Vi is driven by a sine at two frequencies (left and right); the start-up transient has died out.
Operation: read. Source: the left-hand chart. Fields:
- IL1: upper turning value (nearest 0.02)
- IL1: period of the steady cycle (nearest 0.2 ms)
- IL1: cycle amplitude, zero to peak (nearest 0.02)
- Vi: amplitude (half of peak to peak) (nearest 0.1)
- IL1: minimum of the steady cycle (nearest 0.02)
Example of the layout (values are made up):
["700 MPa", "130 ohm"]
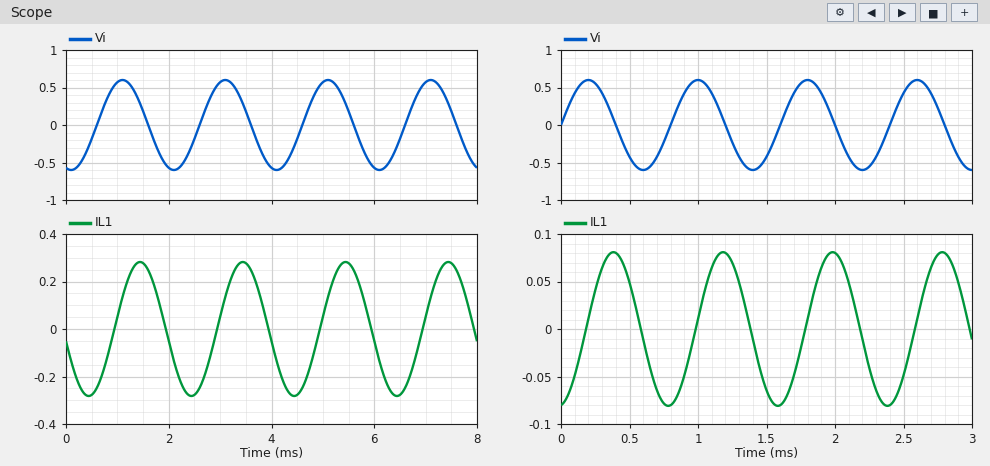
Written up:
["0.28", "2.0 ms", "0.28", "0.6", "-0.28"]
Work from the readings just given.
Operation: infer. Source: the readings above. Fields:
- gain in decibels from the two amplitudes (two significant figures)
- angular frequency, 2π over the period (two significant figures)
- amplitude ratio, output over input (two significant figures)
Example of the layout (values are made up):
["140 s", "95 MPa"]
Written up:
["-6.6 dB", "3.1 rad/ms", "0.47"]
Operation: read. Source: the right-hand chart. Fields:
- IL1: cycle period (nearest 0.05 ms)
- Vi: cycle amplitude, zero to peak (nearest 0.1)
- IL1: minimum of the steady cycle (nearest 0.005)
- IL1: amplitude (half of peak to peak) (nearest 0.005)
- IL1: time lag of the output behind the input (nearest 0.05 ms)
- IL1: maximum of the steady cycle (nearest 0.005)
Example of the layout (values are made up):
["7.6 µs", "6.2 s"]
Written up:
["0.80 ms", "0.6", "-0.080", "0.080", "0.20 ms", "0.080"]
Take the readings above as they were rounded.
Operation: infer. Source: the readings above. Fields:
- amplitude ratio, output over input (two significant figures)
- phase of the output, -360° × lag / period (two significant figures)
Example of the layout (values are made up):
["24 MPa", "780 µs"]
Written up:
["0.13", "-90°"]
